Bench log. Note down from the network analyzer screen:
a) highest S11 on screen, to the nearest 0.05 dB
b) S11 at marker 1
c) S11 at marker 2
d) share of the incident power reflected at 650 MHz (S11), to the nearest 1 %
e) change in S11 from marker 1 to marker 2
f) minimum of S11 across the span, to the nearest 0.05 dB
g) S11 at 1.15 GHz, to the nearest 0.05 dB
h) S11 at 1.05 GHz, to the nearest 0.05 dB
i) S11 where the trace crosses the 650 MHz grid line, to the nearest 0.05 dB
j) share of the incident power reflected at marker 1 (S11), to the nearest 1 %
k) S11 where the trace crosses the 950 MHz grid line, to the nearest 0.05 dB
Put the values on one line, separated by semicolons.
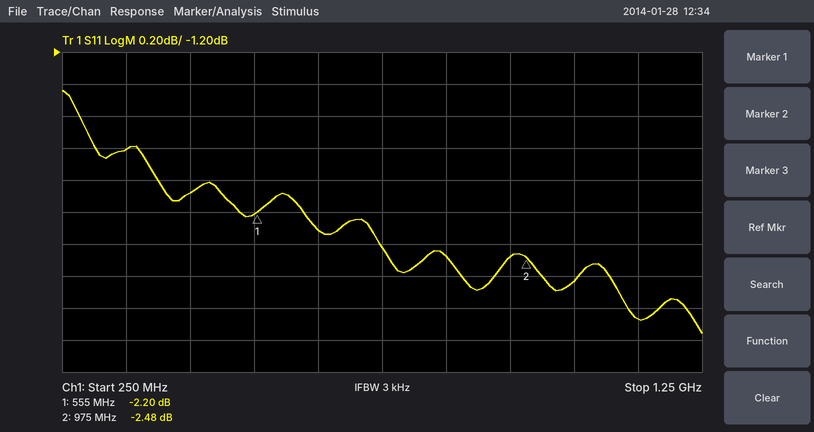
-1.45 dB; -2.20 dB; -2.48 dB; 59 %; -0.28 dB; -2.95 dB; -2.85 dB; -2.65 dB; -2.30 dB; 60 %; -2.50 dB
